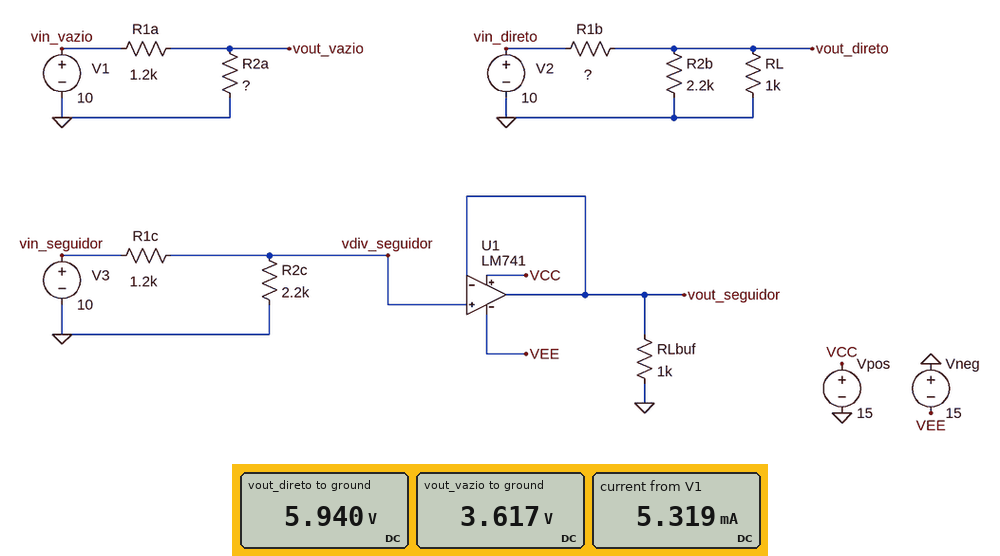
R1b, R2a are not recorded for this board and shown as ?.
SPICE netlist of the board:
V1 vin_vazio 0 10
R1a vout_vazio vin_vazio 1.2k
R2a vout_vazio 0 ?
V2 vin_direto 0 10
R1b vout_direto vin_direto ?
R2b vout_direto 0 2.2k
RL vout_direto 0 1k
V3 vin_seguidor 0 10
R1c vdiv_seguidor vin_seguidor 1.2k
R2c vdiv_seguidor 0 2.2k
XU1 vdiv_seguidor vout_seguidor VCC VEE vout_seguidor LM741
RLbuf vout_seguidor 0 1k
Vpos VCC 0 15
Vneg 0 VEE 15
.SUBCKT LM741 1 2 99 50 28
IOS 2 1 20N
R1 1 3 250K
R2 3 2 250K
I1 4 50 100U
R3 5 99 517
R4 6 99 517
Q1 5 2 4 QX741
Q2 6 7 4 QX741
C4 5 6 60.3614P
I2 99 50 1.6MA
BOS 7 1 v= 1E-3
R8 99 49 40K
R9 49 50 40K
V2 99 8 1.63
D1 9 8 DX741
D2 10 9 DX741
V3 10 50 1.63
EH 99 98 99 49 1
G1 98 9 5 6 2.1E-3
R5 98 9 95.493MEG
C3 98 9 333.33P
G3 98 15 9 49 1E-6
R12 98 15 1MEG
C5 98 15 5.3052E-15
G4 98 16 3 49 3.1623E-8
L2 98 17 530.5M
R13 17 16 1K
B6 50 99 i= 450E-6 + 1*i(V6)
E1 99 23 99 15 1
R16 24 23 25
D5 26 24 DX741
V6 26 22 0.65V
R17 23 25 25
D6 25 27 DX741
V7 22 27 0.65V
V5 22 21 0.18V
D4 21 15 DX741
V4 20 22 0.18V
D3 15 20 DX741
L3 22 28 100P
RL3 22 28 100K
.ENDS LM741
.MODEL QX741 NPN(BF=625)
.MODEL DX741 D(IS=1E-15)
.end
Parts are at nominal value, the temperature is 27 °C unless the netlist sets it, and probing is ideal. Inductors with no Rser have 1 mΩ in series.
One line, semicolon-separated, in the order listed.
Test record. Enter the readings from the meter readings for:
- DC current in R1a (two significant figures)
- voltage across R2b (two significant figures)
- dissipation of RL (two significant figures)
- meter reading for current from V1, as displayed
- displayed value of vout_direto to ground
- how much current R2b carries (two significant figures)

5.3 mA; 5.9 V; 35 mW; 5.319 mA; 5.940 V; 2.7 mA
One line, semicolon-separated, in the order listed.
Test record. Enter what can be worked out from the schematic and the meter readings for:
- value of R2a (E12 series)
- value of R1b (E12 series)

680 Ω; 470 Ω
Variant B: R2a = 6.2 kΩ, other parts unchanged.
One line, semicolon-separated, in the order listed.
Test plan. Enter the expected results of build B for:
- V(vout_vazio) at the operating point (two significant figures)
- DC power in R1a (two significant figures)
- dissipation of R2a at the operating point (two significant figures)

8.4 V; 2.2 mW; 11 mW
